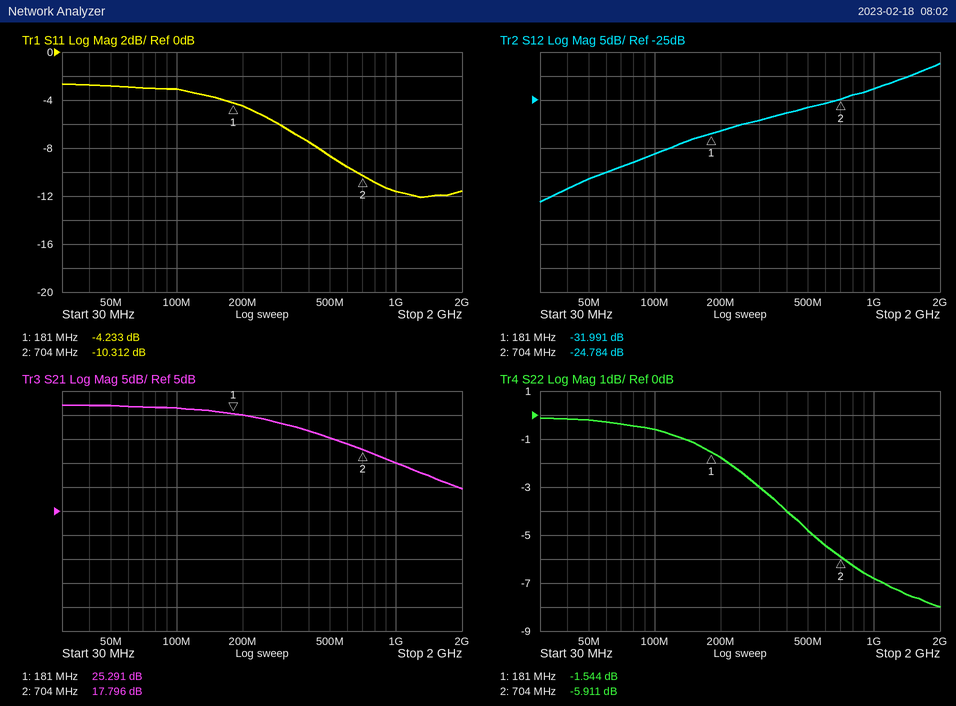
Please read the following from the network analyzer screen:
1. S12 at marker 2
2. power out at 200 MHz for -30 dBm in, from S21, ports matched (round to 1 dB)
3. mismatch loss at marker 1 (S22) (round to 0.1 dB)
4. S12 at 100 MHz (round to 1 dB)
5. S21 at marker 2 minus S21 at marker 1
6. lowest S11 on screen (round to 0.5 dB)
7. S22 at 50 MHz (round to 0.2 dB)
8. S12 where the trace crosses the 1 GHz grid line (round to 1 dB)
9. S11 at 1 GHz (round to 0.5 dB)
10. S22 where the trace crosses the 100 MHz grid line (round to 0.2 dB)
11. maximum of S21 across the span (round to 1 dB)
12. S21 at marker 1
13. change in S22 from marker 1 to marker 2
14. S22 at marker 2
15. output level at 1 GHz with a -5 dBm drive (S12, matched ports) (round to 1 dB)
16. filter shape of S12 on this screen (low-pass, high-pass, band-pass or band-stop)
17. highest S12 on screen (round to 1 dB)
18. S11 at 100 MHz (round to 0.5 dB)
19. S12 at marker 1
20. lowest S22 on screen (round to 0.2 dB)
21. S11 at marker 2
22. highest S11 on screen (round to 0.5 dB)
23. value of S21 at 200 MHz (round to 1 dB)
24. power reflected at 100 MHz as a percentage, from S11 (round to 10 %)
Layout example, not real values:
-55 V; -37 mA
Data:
-24.784 dB; -5 dBm; 5.2 dB; -36 dB; -7.495 dB; -12.0 dB; -0.2 dB; -23 dB; -11.5 dB; -0.6 dB; 27 dB; 25.291 dB; -4.367 dB; -5.911 dB; -28 dBm; high-pass; -17 dB; -3.0 dB; -31.991 dB; -8.0 dB; -10.312 dB; -2.5 dB; 25 dB; 50 %
